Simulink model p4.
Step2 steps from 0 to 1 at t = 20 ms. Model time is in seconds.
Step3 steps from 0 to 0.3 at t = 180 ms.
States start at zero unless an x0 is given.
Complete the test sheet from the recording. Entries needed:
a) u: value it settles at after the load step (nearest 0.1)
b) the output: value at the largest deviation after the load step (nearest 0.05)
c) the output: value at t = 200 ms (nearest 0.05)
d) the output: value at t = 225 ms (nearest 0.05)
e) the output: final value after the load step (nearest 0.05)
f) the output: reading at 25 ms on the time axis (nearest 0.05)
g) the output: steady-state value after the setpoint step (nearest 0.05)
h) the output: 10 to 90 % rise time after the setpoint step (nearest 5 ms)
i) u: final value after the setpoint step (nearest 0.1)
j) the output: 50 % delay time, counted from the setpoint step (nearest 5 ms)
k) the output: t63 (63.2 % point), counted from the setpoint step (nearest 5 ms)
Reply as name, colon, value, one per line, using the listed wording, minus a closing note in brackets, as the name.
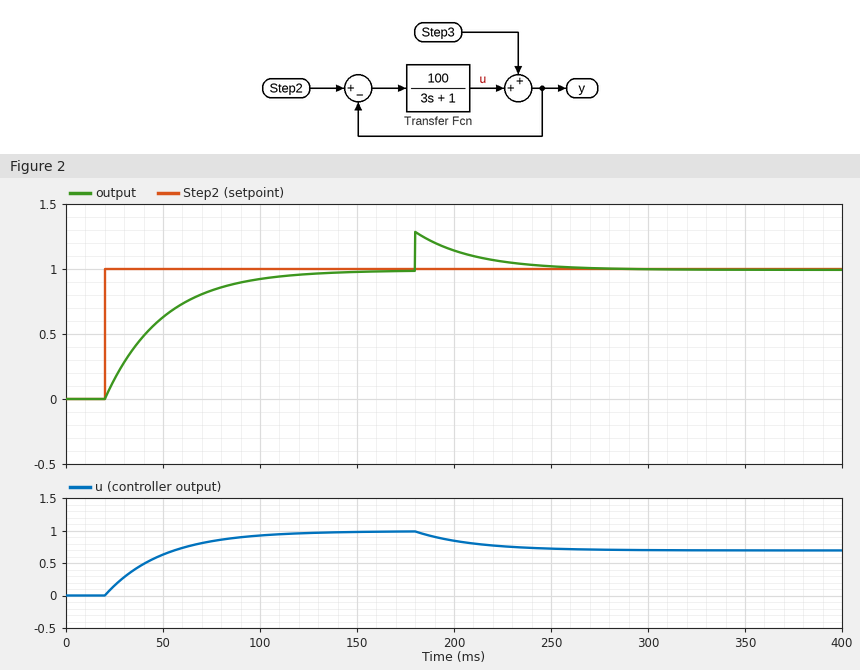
u: value it settles at after the load step: 0.7
the output: value at the largest deviation after the load step: 1.30
the output: value at t = 200 ms: 1.15
the output: value at t = 225 ms: 1.05
the output: final value after the load step: 1.00
the output: reading at 25 ms on the time axis: 0.15
the output: steady-state value after the setpoint step: 1.00
the output: 10 to 90 % rise time after the setpoint step: 65 ms
u: final value after the setpoint step: 1.0
the output: 50 % delay time, counted from the setpoint step: 20 ms
the output: t63 (63.2 % point), counted from the setpoint step: 30 ms
